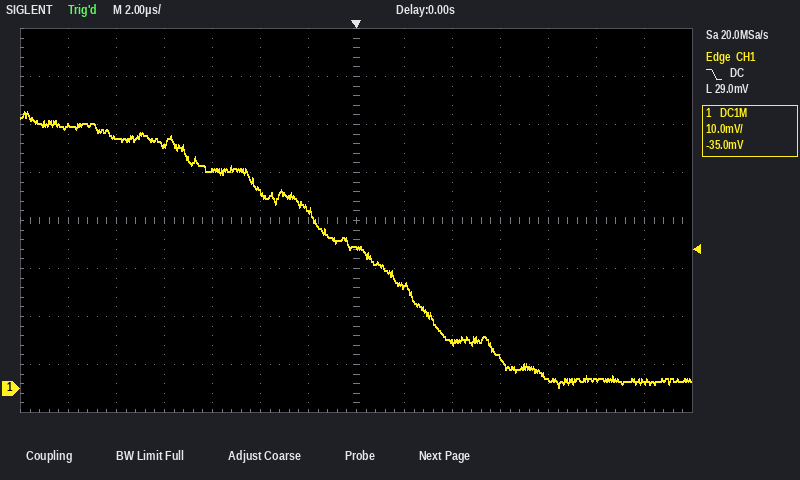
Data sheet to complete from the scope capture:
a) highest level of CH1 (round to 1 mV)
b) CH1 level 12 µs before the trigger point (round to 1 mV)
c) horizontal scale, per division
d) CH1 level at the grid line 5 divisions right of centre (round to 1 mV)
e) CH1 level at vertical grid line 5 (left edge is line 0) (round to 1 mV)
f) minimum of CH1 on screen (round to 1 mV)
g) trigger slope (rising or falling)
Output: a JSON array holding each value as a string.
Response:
["58 mV", "55 mV", "2 µs", "2 mV", "41 mV", "0 mV", "falling"]
